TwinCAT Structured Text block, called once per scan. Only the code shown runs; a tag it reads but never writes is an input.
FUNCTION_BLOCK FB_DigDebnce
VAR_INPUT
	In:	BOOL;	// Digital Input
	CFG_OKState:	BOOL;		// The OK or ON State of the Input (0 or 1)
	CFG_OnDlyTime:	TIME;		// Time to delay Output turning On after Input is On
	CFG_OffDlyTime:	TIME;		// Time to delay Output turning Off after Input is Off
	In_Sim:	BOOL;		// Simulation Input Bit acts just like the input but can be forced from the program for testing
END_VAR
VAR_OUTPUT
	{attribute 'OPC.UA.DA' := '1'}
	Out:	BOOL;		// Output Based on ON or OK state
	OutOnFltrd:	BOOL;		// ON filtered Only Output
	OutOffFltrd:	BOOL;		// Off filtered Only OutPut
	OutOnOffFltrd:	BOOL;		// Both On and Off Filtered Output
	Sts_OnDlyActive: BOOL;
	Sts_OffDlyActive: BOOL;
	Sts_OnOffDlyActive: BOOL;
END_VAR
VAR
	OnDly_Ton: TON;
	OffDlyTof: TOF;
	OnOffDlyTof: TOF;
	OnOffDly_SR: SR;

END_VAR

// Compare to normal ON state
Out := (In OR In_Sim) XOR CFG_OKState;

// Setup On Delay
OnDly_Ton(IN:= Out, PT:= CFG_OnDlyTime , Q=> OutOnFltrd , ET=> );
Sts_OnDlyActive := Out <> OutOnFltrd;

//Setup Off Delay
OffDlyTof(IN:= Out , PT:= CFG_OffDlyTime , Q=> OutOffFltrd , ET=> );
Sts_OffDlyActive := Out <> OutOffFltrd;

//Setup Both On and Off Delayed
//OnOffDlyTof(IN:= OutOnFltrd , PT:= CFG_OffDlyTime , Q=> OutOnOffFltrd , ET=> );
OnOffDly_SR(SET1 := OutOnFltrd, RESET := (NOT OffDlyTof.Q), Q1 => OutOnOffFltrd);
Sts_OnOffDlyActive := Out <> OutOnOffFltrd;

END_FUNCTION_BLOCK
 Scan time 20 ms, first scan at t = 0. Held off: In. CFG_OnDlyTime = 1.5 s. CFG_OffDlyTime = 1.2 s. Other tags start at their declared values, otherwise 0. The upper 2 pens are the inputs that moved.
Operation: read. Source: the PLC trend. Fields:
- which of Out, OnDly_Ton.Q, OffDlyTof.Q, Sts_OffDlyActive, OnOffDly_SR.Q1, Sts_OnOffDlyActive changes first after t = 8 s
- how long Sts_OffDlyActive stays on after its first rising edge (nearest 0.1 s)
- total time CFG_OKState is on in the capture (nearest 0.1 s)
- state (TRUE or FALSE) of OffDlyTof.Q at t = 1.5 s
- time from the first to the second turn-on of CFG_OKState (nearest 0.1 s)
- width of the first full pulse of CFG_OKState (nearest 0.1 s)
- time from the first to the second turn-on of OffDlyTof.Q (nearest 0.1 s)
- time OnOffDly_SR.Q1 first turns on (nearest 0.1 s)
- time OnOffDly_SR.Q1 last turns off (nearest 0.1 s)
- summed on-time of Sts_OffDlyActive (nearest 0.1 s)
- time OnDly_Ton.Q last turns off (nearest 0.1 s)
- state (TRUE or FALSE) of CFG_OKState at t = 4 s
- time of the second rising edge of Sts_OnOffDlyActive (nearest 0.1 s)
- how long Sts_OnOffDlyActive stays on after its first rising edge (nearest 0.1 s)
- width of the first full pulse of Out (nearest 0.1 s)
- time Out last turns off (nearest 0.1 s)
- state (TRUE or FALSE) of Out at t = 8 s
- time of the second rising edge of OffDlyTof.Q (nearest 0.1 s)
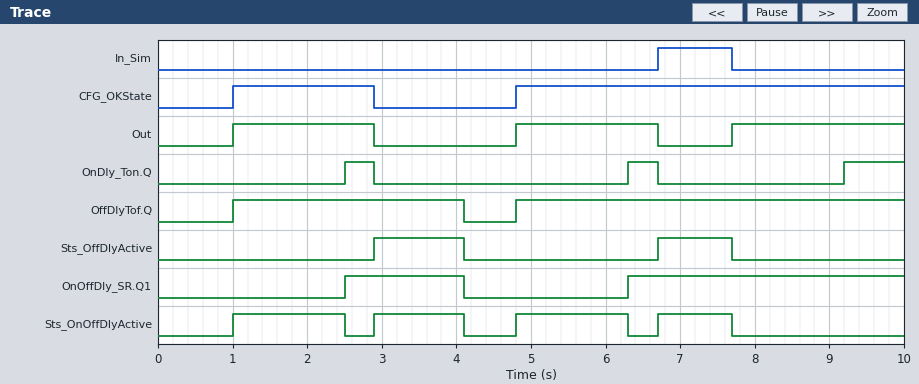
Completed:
OnDly_Ton.Q
1.2 s
7.1 s
TRUE
3.8 s
1.9 s
3.8 s
2.5 s
4.1 s
2.2 s
6.7 s
FALSE
2.9 s
1.5 s
1.9 s
6.7 s
TRUE
4.8 s
